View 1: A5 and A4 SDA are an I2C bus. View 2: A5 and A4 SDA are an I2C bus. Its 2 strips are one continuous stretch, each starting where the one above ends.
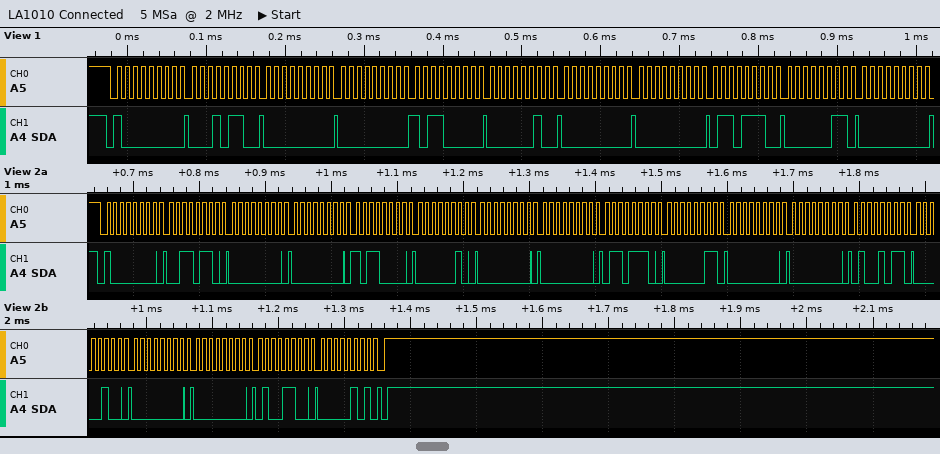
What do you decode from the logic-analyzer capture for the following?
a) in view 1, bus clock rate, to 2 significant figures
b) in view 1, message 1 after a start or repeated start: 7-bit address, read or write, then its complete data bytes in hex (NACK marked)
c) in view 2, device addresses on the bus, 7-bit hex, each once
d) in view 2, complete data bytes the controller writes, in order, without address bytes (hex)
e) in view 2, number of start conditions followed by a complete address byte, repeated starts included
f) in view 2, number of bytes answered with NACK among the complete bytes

100 kHz
0x40 write: 16 00 00 B0 02 00 00 6E 03 00
0x40
36 00 00 B0 02 00 00 6E 03 00 00 4B 04 00 00 4C 05
1
0
